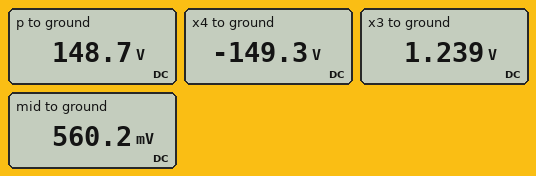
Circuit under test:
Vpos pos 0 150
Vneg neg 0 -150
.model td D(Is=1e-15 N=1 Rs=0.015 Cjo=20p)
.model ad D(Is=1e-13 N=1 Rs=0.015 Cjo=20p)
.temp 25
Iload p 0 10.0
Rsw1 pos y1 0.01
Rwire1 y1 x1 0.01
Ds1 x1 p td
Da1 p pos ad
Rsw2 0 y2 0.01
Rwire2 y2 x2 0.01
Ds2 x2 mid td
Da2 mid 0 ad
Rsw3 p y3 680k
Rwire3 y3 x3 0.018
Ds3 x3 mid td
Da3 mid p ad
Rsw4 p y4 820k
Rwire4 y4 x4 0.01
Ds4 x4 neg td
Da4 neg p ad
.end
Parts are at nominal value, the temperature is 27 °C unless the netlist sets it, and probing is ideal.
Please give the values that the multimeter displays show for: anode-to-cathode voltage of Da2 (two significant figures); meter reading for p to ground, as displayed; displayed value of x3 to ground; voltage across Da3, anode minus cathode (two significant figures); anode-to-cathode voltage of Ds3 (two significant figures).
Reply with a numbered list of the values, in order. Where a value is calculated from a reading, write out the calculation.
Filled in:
1. 560.2 mV = 560 mV
2. 148.7 V
3. 1.239 V
4. 560.2 mV - 148.7 V = -150 V
5. 1.239 V - 560.2 mV = 680 mV
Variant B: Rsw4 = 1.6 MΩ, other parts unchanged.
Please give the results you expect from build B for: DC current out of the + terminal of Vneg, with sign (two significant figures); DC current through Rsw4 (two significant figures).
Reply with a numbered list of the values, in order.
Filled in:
1. -190 µA
2. 190 µA
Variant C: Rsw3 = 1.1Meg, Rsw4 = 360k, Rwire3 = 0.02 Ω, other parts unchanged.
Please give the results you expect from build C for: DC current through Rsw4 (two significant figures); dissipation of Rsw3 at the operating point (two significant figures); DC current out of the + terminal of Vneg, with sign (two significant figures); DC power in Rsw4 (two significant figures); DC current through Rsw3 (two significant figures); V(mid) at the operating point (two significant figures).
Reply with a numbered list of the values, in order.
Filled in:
1. 830 µA
2. 20 mW
3. -830 µA
4. 250 mW
5. 130 µA
6. 550 mV
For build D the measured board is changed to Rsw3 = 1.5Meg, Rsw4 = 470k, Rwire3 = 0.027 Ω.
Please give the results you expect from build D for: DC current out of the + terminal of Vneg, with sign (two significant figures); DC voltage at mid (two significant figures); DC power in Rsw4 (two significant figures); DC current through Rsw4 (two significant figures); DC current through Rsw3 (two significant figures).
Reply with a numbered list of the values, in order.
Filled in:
1. -630 µA
2. 540 mV
3. 190 mW
4. 630 µA
5. 98 µA
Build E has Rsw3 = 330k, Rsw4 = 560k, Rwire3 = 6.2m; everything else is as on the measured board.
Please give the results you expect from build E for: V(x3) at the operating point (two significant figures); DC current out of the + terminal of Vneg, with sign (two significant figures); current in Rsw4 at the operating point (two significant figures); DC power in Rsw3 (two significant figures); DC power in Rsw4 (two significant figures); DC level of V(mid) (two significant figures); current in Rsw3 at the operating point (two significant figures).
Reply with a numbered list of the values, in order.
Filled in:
1. 1.3 V
2. -530 µA
3. 530 µA
4. 66 mW
5. 160 mW
6. 580 mV
7. 450 µA
